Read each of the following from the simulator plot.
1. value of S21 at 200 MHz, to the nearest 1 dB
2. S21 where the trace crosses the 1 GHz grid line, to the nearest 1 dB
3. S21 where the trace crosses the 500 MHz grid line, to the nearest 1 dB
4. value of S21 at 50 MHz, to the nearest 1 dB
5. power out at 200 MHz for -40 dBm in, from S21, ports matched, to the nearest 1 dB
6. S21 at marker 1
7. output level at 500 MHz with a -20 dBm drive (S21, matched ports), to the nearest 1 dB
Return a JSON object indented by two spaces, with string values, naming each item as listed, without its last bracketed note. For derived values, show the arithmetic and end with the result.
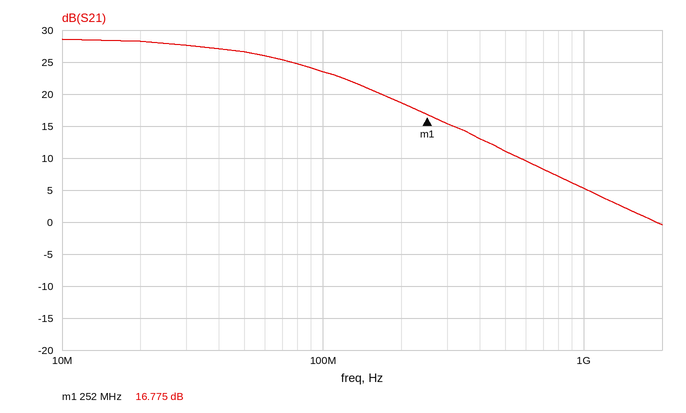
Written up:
{
  "value of S21 at 200 MHz, to the nearest 1 dB": "19 dB",
  "S21 where the trace crosses the 1 GHz grid line, to the nearest 1 dB": "5 dB",
  "S21 where the trace crosses the 500 MHz grid line, to the nearest 1 dB": "11 dB",
  "value of S21 at 50 MHz, to the nearest 1 dB": "27 dB",
  "power out at 200 MHz for -40 dBm in, from S21, ports matched, to the nearest 1 dB": "-40 dBm + (19 dB) = -21 dBm",
  "S21 at marker 1": "16.775 dB",
  "output level at 500 MHz with a -20 dBm drive (S21, matched ports), to the nearest 1 dB": "-20 dBm + (11 dB) = -9 dBm"
}
